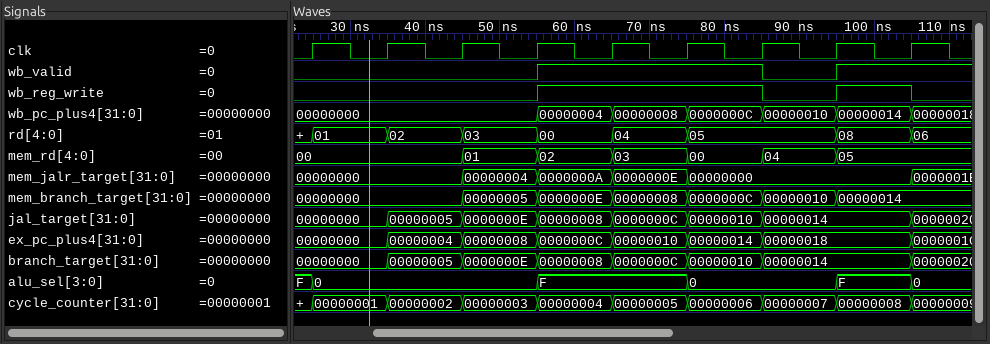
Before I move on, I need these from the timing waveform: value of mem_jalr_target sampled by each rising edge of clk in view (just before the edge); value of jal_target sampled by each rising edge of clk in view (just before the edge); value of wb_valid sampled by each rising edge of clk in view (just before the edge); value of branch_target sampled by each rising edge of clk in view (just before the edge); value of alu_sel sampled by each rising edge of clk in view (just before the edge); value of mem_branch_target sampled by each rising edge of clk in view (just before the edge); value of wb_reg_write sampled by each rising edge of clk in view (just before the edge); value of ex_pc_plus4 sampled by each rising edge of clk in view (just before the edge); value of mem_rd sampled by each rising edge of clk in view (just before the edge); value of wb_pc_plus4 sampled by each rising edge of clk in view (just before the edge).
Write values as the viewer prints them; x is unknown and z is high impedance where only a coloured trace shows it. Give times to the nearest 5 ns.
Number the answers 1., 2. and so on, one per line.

1. 00000000, 00000000, 00000000, 00000004, 0000000A, 0000000E, 00000000, 00000000, 00000000
2. 00000000, 00000000, 00000005, 0000000E, 00000008, 0000000C, 00000010, 00000014, 00000014
3. 0 0 0 0 1 1 1 0 1
4. 00000000, 00000000, 00000005, 0000000E, 00000008, 0000000C, 00000010, 00000014, 00000014
5. F, 0, 0, 0, F, F, 0, 0, F
6. 00000000, 00000000, 00000000, 00000005, 0000000E, 00000008, 0000000C, 00000010, 00000014
7. 0 0 0 0 1 1 1 0 1
8. 00000000, 00000000, 00000004, 00000008, 0000000C, 00000010, 00000014, 00000018, 00000018
9. 00, 00, 00, 01, 02, 03, 00, 04, 05
10. 00000000, 00000000, 00000000, 00000000, 00000004, 00000008, 0000000C, 00000010, 00000014
